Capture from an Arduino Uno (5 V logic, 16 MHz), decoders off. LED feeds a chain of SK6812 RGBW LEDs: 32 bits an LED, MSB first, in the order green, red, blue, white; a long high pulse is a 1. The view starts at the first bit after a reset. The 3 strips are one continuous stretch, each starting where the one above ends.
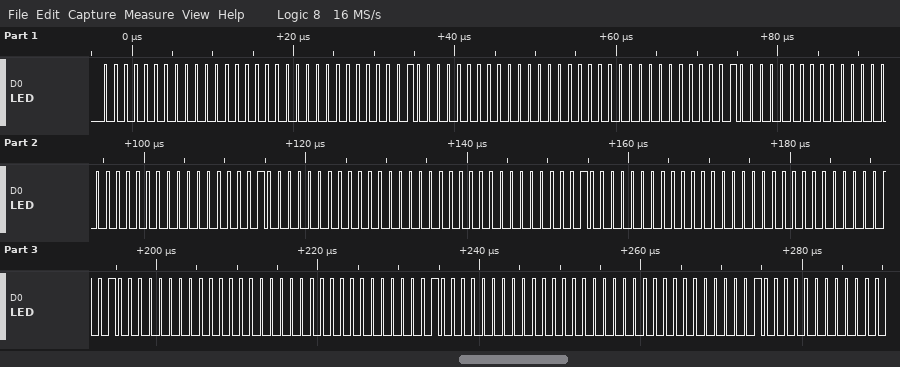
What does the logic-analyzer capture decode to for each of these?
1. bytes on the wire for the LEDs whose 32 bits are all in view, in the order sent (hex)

00 00 00 02 00 00 00 02 00 00 00 02 00 00 00 02 00 00 00 02 00 00 00 02 00 00 00 02
